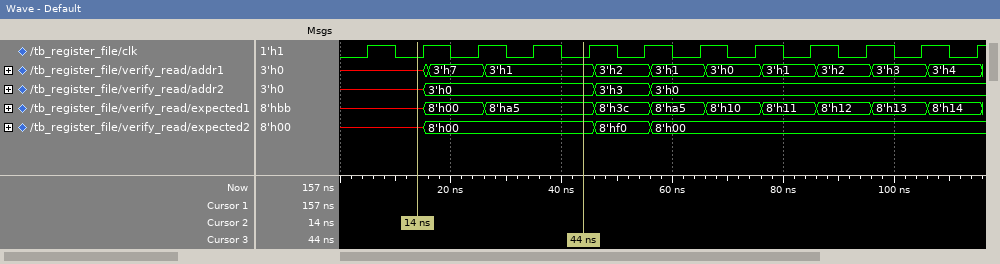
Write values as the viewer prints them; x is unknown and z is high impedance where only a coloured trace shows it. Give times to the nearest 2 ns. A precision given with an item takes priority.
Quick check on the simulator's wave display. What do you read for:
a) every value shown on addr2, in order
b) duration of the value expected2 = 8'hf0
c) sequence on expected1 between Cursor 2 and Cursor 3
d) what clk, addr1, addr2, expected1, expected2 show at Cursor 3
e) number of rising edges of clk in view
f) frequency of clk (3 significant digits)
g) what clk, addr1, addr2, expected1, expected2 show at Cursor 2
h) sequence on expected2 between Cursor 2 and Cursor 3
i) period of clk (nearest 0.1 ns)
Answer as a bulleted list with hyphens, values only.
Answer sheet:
- x, 3'h0, 3'h3, 3'h0
- 10 ns
- x, 8'h00, 8'ha5
- clk=0, addr1=3'h1, addr2=3'h0, expected1=8'ha5, expected2=8'h00
- 12
- 100 MHz
- clk=0, addr1=x, addr2=x, expected1=x, expected2=x
- x, 8'h00
- 10 ns
